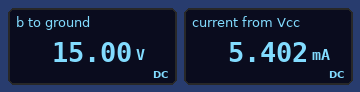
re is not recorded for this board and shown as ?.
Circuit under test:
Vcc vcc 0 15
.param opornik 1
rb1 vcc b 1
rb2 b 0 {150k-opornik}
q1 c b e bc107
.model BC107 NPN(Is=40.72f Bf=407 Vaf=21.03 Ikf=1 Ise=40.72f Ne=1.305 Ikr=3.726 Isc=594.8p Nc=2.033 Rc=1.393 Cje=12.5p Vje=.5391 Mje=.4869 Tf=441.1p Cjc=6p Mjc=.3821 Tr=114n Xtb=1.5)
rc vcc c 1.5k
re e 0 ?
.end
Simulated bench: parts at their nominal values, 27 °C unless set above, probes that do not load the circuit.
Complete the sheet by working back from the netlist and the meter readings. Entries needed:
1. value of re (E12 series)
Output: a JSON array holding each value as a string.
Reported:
["2.7 kΩ"]
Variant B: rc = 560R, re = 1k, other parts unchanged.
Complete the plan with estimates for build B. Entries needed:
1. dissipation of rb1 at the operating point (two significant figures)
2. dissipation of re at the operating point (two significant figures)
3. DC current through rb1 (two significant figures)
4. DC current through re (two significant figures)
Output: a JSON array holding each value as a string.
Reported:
["170 µW", "200 mW", "13 mA", "14 mA"]
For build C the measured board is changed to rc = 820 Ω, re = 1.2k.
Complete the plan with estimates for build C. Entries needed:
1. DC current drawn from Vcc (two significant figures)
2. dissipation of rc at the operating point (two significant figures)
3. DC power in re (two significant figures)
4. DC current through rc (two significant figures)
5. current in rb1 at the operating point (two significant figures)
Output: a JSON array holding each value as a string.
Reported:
["12 mA", "580 µW", "170 mW", "840 µA", "11 mA"]
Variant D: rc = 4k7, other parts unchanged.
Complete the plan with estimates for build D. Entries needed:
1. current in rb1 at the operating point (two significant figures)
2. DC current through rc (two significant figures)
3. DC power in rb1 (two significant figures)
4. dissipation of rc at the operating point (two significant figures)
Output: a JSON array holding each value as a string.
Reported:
["5.3 mA", "140 µA", "28 µW", "94 µW"]
